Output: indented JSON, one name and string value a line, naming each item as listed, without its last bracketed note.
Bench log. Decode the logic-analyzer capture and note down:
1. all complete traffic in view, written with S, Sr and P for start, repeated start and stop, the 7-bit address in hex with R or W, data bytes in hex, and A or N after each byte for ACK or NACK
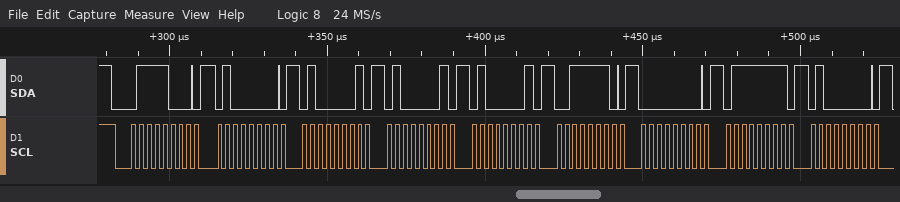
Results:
{
  "all complete traffic in view, written with S, Sr and P for start, repeated start and stop, the 7-bit address in hex with R or W, data bytes in hex, and A or N after each byte for ACK or NACK": "S 3CW A 40 A 41 A 41 A 41 A 3E A 00 A 7F A 40 A"
}
